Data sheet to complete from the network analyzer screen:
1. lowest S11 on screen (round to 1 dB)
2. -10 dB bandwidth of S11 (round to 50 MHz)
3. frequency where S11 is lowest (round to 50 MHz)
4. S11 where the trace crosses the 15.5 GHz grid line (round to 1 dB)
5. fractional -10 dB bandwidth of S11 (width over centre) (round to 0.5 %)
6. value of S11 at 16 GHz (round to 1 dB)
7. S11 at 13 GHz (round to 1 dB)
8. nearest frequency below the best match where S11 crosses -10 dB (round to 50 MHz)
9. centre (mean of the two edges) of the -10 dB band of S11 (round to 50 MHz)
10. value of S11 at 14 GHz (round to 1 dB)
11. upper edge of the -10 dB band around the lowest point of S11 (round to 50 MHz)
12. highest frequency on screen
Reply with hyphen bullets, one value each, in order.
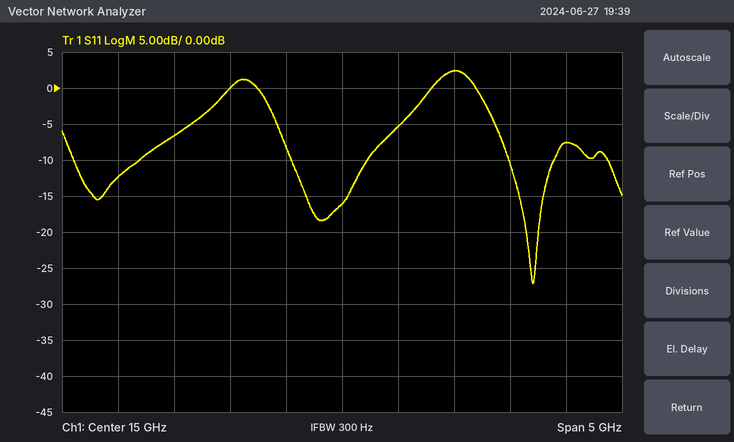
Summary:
- -27 dB
- 400 MHz
- 16.70 GHz
- -5 dB
- 2.5 %
- 2 dB
- -12 dB
- 16.50 GHz
- 16.70 GHz
- 0 dB
- 16.90 GHz
- 17.5 GHz
